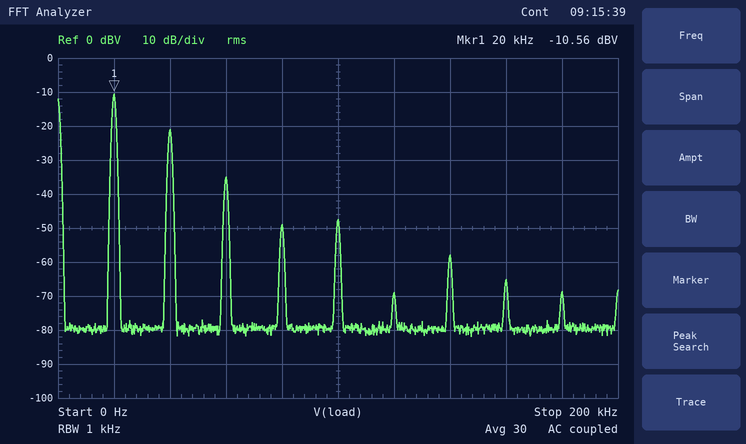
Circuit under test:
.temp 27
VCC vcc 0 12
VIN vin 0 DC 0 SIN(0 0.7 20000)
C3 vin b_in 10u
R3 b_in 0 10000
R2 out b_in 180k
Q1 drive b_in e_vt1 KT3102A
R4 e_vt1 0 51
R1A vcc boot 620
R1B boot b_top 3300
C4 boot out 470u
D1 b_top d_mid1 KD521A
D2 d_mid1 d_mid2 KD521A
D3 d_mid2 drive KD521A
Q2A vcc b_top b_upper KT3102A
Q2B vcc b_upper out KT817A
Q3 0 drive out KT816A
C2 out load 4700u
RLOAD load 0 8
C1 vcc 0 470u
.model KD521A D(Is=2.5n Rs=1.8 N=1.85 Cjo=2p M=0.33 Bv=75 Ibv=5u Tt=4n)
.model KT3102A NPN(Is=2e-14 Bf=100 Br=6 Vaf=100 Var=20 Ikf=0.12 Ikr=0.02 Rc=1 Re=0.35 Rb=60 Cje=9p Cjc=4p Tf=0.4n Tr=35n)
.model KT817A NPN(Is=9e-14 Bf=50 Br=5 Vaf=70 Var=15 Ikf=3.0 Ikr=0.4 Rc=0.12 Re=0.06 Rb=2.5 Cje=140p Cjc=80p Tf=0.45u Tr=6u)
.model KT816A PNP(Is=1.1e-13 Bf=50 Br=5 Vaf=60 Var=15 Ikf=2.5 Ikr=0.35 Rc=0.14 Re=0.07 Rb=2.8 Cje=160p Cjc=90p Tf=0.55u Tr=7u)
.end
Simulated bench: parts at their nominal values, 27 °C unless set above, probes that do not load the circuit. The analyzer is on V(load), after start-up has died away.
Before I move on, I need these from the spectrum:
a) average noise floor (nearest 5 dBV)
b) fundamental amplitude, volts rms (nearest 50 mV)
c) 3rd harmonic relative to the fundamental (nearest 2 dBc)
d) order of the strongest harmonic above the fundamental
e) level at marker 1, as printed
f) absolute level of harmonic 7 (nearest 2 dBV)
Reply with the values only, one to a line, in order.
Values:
-80 dBV
300 mV
-24 dBc
2
-10.56 dBV
-58 dBV
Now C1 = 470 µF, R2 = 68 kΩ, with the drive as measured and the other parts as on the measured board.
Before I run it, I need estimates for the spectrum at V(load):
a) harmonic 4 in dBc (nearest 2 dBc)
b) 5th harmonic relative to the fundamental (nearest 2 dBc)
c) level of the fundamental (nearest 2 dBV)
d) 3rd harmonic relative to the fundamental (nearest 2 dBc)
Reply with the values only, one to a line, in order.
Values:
-34 dBc
-42 dBc
-8 dBV
-30 dBc
